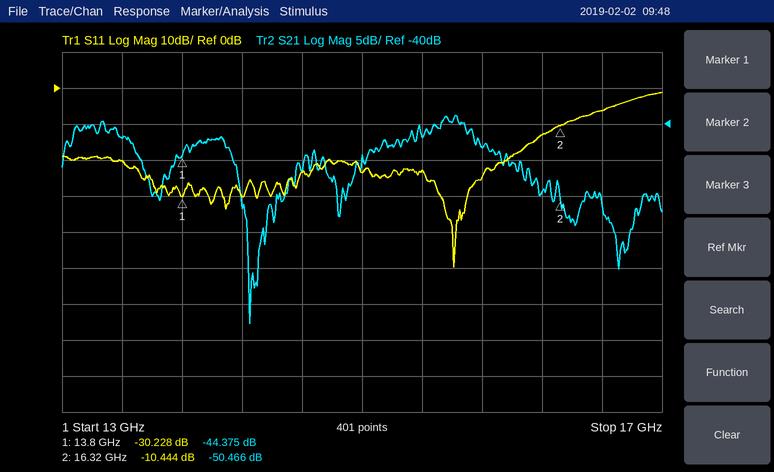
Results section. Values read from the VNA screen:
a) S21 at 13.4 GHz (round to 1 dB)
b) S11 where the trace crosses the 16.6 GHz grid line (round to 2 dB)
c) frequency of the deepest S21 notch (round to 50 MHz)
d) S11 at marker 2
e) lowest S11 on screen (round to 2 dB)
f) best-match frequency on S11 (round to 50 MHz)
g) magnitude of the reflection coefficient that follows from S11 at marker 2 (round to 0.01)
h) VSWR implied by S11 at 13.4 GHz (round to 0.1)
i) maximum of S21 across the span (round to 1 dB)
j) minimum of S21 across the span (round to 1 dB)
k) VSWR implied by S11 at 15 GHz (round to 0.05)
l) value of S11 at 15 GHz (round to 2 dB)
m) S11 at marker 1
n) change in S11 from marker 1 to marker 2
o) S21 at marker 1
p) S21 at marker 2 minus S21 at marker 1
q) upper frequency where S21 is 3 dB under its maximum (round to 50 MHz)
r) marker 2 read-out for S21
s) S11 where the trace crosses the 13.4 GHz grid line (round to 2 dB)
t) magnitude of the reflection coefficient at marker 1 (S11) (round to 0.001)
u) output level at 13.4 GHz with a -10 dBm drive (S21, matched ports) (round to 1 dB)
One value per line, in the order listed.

-42 dB
-6 dB
14.25 GHz
-10.444 dB
-50 dB
15.60 GHz
0.30
1.2
-39 dB
-68 dB
1.15
-24 dB
-30.228 dB
19.784 dB
-44.375 dB
-6.091 dB
15.75 GHz
-50.466 dB
-20 dB
0.031
-52 dBm
